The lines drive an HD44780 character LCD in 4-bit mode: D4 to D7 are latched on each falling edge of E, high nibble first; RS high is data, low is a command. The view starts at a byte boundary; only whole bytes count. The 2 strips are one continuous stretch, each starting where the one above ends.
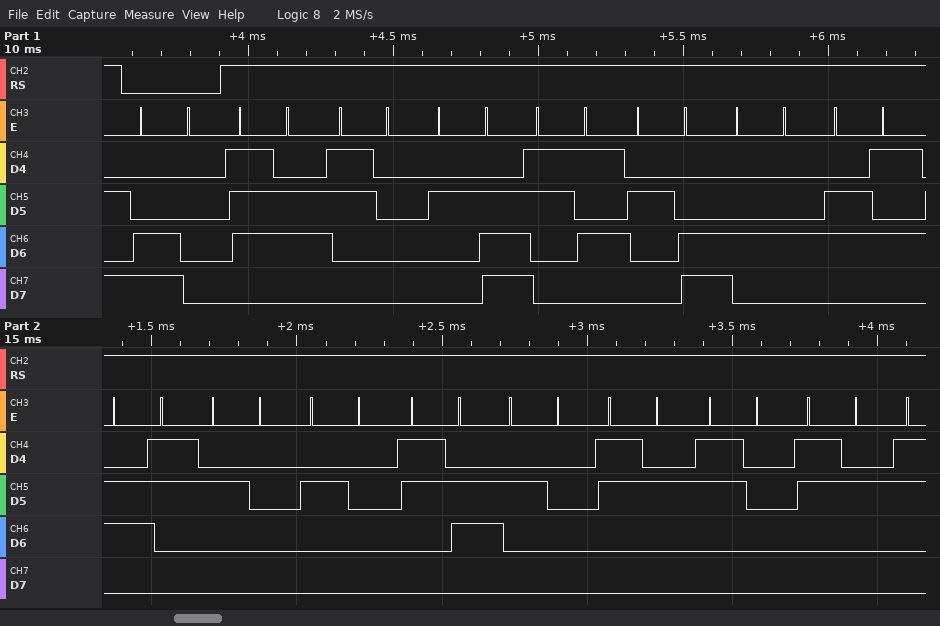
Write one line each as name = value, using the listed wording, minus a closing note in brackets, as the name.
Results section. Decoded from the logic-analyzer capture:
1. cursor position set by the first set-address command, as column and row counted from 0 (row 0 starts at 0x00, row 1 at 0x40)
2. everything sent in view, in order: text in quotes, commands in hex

cursor position set by the first set-address command, as column and row counted from 0 = column 0, row 1
everything sent in view, in order: text in quotes, commands in hex = 0xC0 "v0.5,Dec  6 202"
